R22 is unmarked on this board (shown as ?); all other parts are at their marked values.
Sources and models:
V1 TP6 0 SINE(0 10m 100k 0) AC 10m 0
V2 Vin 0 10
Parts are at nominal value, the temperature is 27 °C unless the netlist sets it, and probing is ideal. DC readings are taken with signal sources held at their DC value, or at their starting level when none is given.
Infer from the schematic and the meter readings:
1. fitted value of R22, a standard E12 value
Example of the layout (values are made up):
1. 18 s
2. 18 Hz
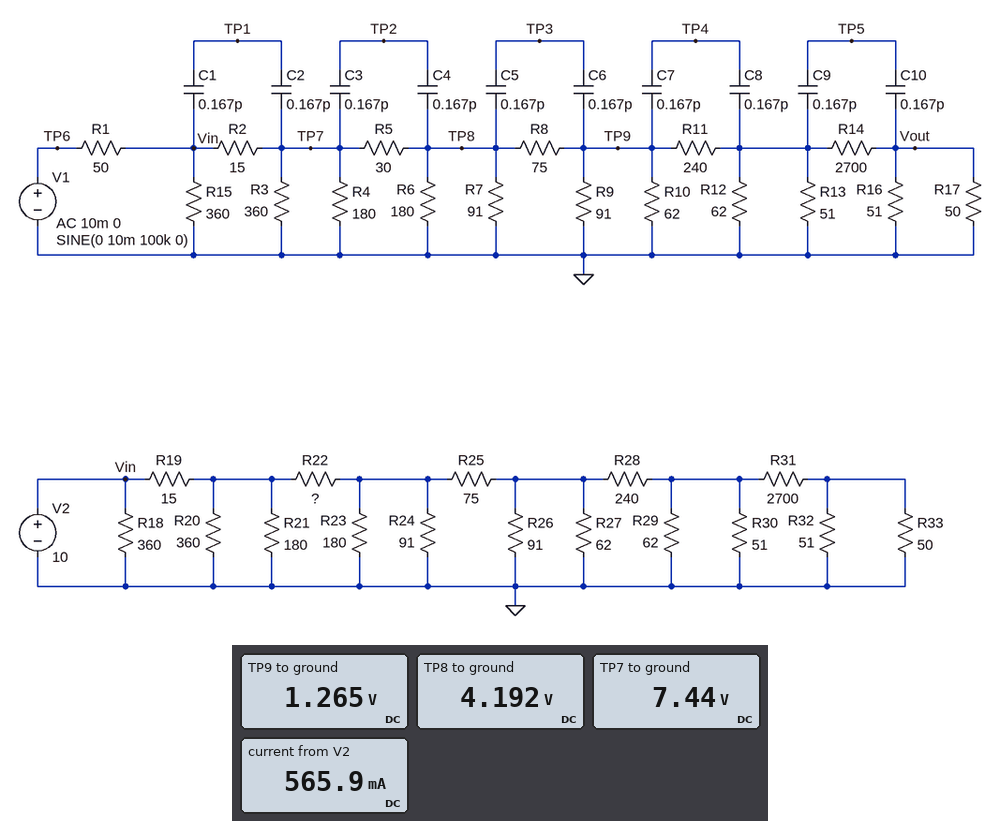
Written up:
1. 68 Ω
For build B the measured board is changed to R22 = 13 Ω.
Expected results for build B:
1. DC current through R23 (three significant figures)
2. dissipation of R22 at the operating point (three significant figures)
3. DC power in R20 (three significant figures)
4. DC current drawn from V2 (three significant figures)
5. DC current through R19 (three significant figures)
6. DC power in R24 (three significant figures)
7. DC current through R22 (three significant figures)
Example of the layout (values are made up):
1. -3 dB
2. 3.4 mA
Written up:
1. 29.4 mA
2. 243 mW
3. 139 mW
4. 622 mA
5. 196 mA
6. 307 mW
7. 137 mA
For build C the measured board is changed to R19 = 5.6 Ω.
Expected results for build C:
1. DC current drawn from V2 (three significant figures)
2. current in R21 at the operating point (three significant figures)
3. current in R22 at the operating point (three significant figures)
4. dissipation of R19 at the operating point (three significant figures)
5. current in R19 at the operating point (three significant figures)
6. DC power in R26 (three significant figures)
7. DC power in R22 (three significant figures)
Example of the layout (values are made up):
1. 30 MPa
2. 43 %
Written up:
1. 587 mA
2. 50.5 mA
3. 85.3 mA
4. 145 mW
5. 161 mA
6. 10.9 mW
7. 495 mW
